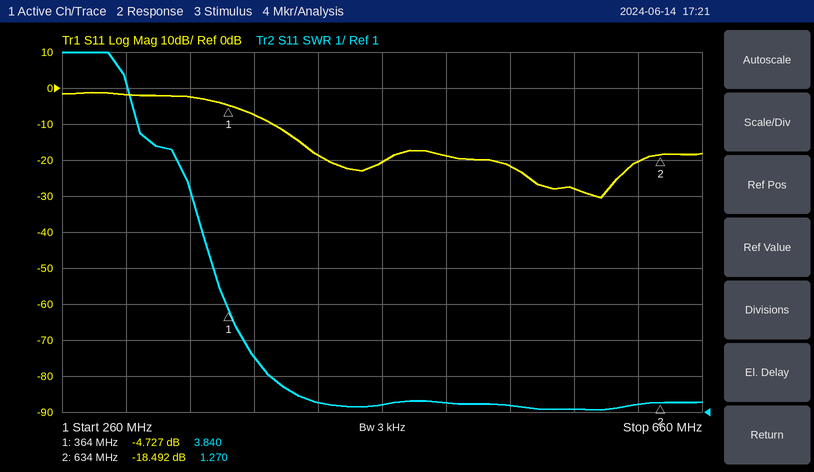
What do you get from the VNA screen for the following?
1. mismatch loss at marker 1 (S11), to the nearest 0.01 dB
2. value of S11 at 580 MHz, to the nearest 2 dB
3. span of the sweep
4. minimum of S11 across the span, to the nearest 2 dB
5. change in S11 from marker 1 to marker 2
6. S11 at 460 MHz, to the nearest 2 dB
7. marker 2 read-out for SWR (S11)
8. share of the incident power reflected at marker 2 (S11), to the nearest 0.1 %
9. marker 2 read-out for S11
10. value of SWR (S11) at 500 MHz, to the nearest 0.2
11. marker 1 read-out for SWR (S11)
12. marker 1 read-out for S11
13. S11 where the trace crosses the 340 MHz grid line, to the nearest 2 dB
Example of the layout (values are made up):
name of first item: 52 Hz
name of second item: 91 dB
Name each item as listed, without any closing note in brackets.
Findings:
mismatch loss at marker 1 (S11), to the nearest 0.01 dB: 1.78 dB
value of S11 at 580 MHz, to the nearest 2 dB: -28 dB
span of the sweep: 400 MHz
minimum of S11 across the span, to the nearest 2 dB: -30 dB
change in S11 from marker 1 to marker 2: -13.765 dB
S11 at 460 MHz, to the nearest 2 dB: -20 dB
marker 2 read-out for SWR: 1.270
share of the incident power reflected at marker 2 (S11), to the nearest 0.1 %: 1.4 %
marker 2 read-out for S11: -18.492 dB
value of SWR (S11) at 500 MHz, to the nearest 0.2: 1.2
marker 1 read-out for SWR: 3.840
marker 1 read-out for S11: -4.727 dB
S11 where the trace crosses the 340 MHz grid line, to the nearest 2 dB: -2 dB
